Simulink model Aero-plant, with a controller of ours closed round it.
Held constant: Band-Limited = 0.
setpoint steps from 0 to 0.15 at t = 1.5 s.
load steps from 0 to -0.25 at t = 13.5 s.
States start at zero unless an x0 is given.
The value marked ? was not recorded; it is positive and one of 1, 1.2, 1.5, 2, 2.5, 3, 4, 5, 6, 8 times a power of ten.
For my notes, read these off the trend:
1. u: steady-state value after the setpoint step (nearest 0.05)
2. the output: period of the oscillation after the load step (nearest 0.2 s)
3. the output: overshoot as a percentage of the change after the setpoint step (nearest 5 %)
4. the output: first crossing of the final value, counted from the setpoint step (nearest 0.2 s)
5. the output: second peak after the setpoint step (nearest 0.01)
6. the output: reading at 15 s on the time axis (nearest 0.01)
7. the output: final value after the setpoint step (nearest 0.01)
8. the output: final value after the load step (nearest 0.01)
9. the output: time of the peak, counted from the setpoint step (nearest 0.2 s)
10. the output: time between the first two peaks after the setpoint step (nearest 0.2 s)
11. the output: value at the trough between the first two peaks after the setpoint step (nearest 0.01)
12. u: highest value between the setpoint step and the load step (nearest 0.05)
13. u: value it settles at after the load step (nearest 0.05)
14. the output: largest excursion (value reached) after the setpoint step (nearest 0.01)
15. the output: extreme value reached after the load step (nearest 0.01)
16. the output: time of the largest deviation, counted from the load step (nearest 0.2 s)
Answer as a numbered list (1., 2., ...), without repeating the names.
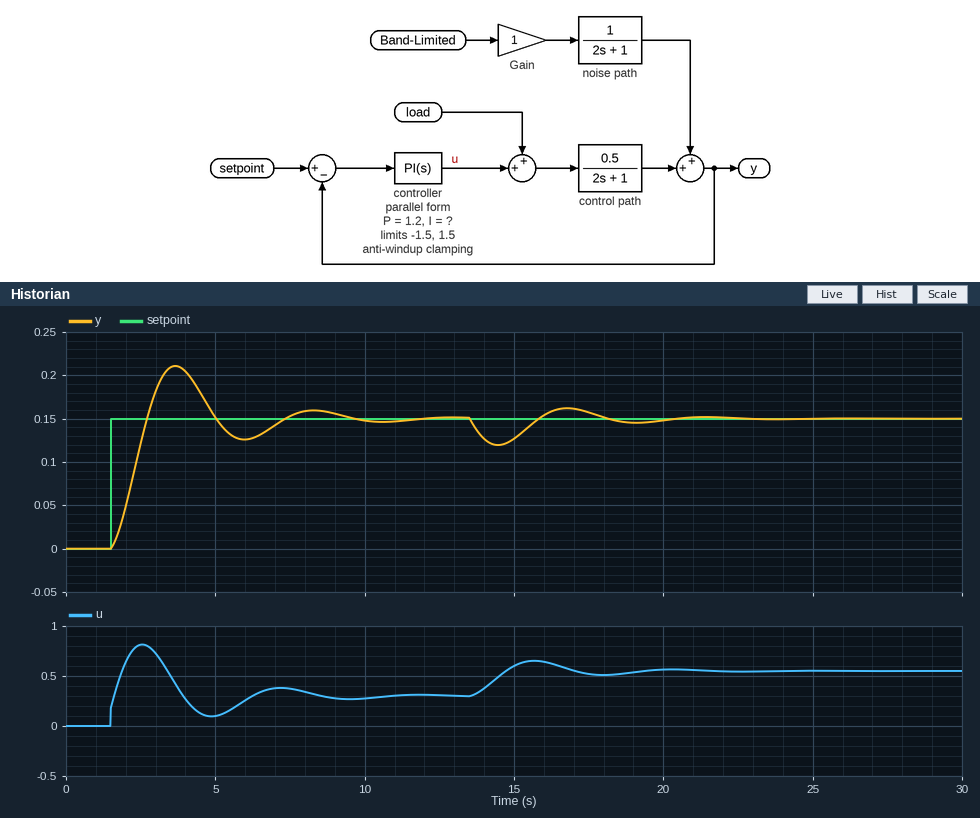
1. 0.30
2. 4.6 s
3. 40 %
4. 1.2 s
5. 0.16
6. 0.13
7. 0.15
8. 0.15
9. 2.2 s
10. 4.6 s
11. 0.13
12. 0.80
13. 0.55
14. 0.21
15. 0.12
16. 1.0 s
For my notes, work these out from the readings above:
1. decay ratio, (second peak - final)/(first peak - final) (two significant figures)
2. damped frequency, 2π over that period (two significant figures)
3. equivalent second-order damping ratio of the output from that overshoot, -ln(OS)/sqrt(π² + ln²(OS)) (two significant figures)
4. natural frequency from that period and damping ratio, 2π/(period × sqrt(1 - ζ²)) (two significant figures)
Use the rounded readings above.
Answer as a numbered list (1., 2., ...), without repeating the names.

1. 0.17
2. 1.4 rad/s
3. 0.28
4. 1.4 rad/s
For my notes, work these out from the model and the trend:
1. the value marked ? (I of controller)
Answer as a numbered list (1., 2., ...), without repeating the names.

1. 8
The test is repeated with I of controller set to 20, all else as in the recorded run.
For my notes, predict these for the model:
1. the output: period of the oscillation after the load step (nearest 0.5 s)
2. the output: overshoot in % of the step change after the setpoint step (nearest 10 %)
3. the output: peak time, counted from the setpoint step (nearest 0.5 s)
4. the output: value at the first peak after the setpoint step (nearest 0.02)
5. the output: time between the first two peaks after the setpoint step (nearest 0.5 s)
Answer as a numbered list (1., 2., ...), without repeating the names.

1. 3.0 s
2. 60 %
3. 1.5 s
4. 0.24
5. 3.0 s
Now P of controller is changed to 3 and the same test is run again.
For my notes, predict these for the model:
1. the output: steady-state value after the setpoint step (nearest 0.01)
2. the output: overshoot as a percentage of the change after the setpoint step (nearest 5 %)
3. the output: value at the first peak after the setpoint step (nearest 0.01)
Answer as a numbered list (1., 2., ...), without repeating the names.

1. 0.15
2. 25 %
3. 0.19
